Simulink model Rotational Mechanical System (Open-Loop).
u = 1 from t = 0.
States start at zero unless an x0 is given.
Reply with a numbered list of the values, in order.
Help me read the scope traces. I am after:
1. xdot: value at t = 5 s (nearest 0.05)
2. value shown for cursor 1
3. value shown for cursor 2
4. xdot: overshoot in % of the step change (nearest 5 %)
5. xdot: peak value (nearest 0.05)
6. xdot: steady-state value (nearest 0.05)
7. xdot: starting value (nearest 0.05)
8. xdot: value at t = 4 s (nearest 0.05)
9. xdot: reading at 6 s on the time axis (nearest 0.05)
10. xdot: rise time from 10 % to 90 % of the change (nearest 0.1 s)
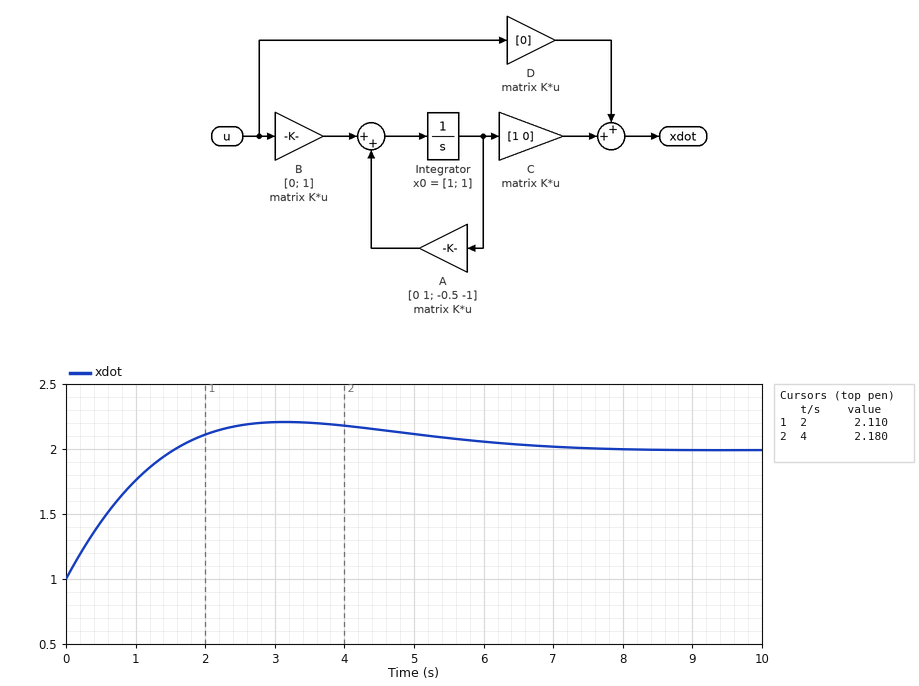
1. 2.10
2. 2.110
3. 2.180
4. 20 %
5. 2.20
6. 2.00
7. 1.00
8. 2.20
9. 2.05
10. 1.2 s
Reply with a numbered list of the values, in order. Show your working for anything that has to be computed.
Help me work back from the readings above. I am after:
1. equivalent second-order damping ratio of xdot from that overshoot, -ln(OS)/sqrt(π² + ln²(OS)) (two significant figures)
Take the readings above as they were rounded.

1. ln(0.2) = -1.609; 1.609 / sqrt(9.870 + 2.590) = 0.46
